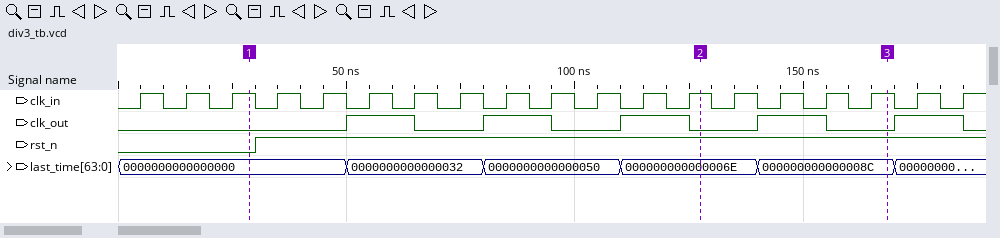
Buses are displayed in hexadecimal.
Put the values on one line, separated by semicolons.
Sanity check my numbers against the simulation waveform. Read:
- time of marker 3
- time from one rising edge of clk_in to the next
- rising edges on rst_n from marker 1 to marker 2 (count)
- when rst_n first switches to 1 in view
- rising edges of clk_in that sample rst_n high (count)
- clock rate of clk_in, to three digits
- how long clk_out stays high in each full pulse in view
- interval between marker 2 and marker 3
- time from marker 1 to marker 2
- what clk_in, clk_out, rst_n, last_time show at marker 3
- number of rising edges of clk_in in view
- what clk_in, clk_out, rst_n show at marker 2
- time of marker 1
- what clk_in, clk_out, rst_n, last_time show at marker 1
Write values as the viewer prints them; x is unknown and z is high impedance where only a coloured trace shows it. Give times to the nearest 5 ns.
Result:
170 ns; 10 ns; 1; 30 ns; 16; 100 MHz; 15 ns, 15 ns, 15 ns, 15 ns, 15 ns; 40 ns; 100 ns; clk_in=1, clk_out=0, rst_n=1, last_time=000000000000008C; 19; clk_in=1, clk_out=0, rst_n=1; 30 ns; clk_in=1, clk_out=0, rst_n=0, last_time=0000000000000000
